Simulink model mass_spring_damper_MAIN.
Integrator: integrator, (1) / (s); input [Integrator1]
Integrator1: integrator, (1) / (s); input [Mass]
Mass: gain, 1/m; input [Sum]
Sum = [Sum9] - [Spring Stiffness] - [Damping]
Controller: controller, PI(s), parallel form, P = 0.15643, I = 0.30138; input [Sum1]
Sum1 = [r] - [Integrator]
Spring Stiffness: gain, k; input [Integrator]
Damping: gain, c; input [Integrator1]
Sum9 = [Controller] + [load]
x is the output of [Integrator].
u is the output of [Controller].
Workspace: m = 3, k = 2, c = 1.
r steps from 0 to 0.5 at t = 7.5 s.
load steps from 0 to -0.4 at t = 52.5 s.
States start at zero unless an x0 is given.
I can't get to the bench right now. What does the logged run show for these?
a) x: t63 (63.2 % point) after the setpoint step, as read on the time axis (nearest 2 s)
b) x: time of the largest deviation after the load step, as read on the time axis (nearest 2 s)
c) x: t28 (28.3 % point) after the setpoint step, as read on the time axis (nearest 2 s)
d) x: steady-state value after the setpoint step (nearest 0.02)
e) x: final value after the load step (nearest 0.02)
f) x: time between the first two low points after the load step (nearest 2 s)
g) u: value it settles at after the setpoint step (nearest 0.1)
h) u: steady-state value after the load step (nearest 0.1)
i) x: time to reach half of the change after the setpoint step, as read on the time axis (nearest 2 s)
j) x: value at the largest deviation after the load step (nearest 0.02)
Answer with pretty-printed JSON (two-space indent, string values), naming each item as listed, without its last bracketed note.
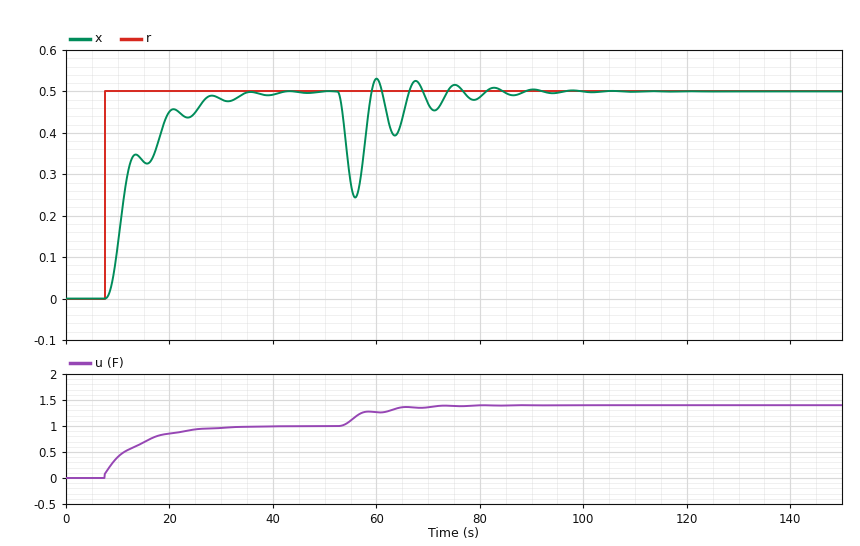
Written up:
{
  "x: t63 (63.2 % point) after the setpoint step, as read on the time axis": "12 s",
  "x: time of the largest deviation after the load step, as read on the time axis": "56 s",
  "x: t28 (28.3 % point) after the setpoint step, as read on the time axis": "10 s",
  "x: steady-state value after the setpoint step": "0.50",
  "x: final value after the load step": "0.50",
  "x: time between the first two low points after the load step": "8 s",
  "u: value it settles at after the setpoint step": "1.0",
  "u: steady-state value after the load step": "1.4",
  "x: time to reach half of the change after the setpoint step, as read on the time axis": "12 s",
  "x: value at the largest deviation after the load step": "0.24"
}
